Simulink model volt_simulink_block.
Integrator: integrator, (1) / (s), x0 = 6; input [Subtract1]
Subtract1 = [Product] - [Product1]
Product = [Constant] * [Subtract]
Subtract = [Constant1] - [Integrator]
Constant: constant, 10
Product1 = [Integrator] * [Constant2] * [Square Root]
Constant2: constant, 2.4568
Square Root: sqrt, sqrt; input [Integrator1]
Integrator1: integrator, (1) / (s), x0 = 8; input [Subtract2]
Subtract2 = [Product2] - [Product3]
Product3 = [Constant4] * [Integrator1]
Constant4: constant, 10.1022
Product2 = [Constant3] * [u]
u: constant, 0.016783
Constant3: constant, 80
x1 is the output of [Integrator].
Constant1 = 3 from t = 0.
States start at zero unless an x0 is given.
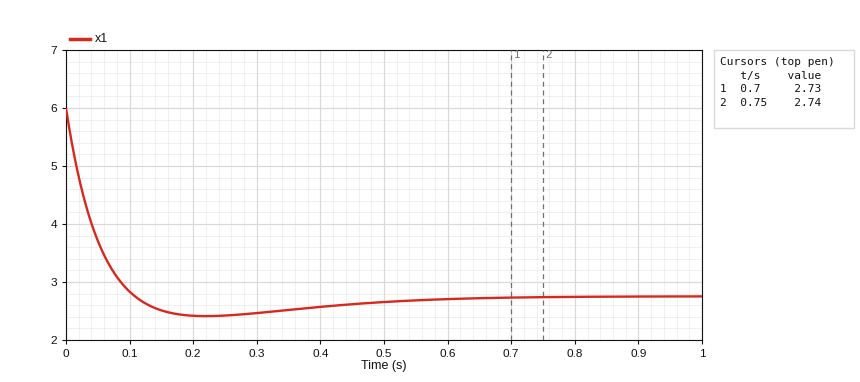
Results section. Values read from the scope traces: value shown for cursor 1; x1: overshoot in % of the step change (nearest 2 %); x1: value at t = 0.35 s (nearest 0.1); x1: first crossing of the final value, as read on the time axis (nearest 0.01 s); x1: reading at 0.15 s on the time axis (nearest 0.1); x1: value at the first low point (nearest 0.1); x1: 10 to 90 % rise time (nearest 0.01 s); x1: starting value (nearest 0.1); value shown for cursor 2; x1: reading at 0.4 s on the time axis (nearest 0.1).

2.73
10 %
2.5
0.11 s
2.5
2.4
0.08 s
6.0
2.74
2.6
